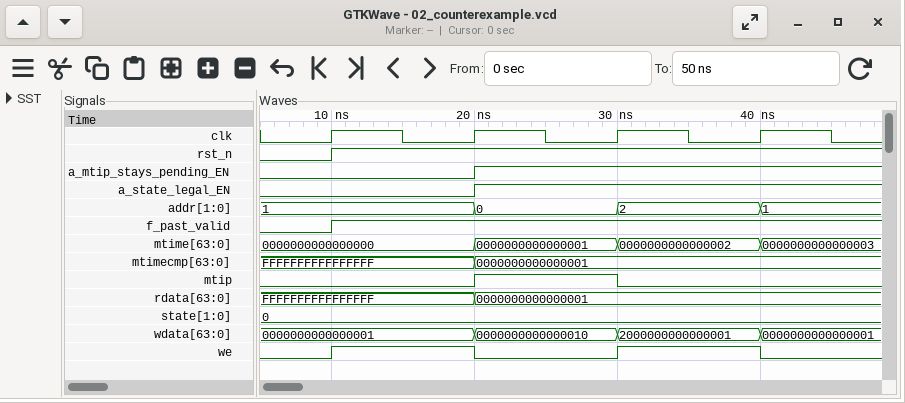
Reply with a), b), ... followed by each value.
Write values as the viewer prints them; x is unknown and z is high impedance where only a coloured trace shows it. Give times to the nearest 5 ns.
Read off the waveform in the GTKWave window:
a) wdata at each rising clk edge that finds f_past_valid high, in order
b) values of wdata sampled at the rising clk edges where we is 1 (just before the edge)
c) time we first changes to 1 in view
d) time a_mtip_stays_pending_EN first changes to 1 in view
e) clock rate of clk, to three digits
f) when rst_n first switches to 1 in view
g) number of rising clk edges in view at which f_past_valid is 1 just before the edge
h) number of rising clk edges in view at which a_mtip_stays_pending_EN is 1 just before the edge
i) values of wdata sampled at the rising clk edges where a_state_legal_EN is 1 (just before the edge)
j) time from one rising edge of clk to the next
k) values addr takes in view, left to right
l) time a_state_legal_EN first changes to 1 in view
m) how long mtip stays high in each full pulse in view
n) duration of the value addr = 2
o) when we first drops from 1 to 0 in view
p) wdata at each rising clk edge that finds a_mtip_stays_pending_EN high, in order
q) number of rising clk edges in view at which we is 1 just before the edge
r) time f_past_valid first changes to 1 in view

a) 0000000000000001, 0000000000000010, 2000000000000001
b) 0000000000000001, 2000000000000001
c) 10 ns
d) 20 ns
e) 100 MHz
f) 10 ns
g) 3
h) 2
i) 0000000000000010, 2000000000000001
j) 10 ns
k) 1, 0, 2, 1
l) 20 ns
m) 10 ns
n) 10 ns
o) 20 ns
p) 0000000000000010, 2000000000000001
q) 2
r) 10 ns
